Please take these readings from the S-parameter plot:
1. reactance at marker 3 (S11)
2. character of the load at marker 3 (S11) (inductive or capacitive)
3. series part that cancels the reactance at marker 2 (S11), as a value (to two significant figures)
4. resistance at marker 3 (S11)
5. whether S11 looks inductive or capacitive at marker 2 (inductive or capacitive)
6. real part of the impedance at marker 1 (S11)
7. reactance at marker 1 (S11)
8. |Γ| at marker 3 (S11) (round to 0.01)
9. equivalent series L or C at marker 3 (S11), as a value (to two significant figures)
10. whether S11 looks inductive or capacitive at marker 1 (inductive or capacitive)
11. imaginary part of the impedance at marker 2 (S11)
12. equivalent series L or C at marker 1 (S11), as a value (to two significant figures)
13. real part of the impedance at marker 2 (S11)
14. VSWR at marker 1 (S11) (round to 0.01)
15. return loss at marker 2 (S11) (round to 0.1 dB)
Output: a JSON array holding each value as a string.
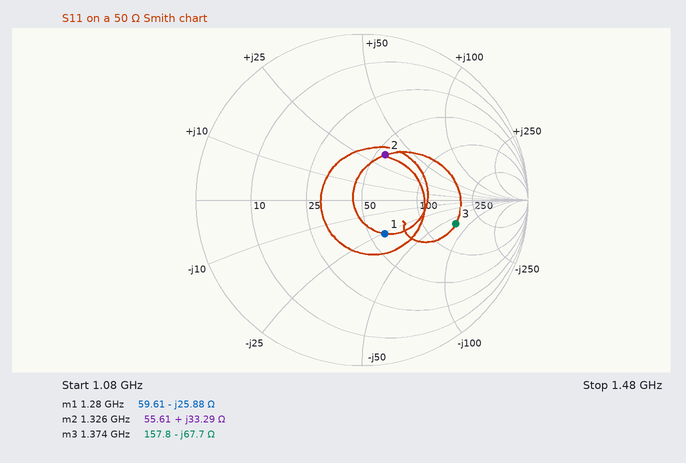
["-67.7 Ω", "capacitive", "3.6 pF", "157.8 Ω", "inductive", "59.61 Ω", "-25.88 Ω", "0.58", "1.7 pF", "capacitive", "+33.29 Ω", "4.8 pF", "55.61 Ω", "1.65", "10.3 dB"]
